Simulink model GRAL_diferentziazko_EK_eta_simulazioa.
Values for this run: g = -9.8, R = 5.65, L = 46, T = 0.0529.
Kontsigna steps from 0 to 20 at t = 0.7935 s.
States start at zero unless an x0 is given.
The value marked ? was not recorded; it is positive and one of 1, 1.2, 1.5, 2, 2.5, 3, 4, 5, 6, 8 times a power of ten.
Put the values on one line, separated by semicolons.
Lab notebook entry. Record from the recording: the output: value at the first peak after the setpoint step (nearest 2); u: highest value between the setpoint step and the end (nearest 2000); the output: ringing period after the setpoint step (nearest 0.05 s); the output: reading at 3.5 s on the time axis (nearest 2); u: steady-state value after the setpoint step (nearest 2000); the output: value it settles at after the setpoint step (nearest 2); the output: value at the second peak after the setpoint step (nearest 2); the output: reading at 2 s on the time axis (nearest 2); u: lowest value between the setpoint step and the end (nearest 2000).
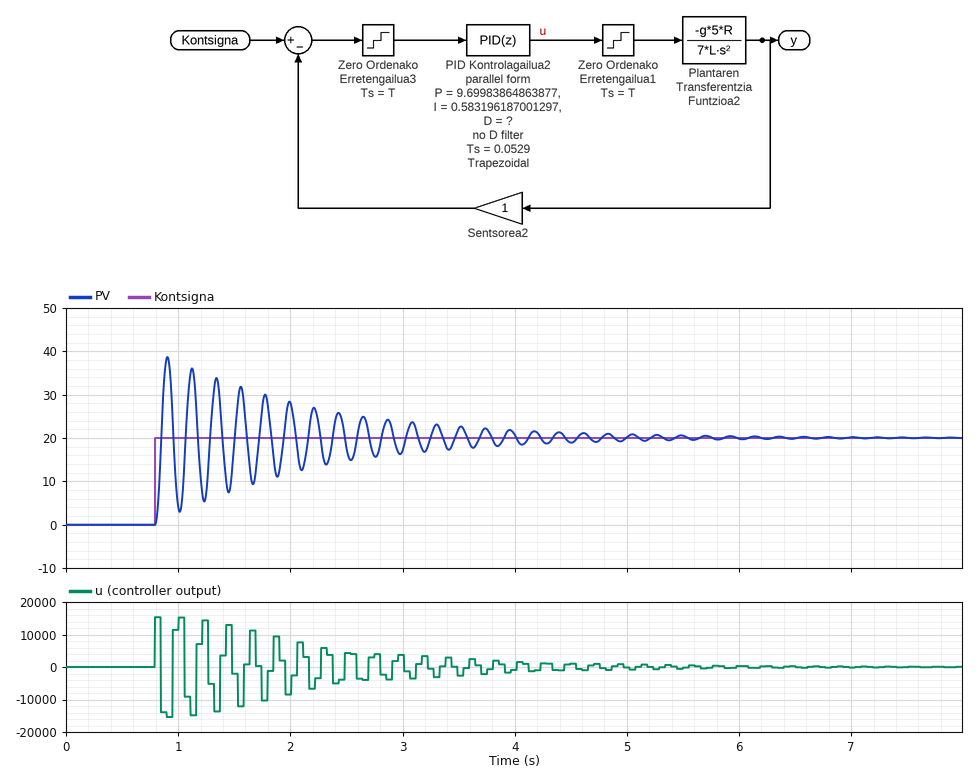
38; 16000; 0.20 s; 22; 0; 20; 36; 28; -16000
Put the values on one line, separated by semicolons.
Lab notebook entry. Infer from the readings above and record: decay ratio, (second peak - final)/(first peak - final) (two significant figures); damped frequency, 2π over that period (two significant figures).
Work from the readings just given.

0.89; 31 rad/s
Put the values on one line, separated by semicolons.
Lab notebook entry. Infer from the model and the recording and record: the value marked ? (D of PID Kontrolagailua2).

40
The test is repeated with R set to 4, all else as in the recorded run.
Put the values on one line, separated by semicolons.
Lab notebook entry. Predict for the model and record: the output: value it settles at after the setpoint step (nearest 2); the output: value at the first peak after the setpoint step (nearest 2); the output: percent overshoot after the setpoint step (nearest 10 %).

20; 32; 60 %
